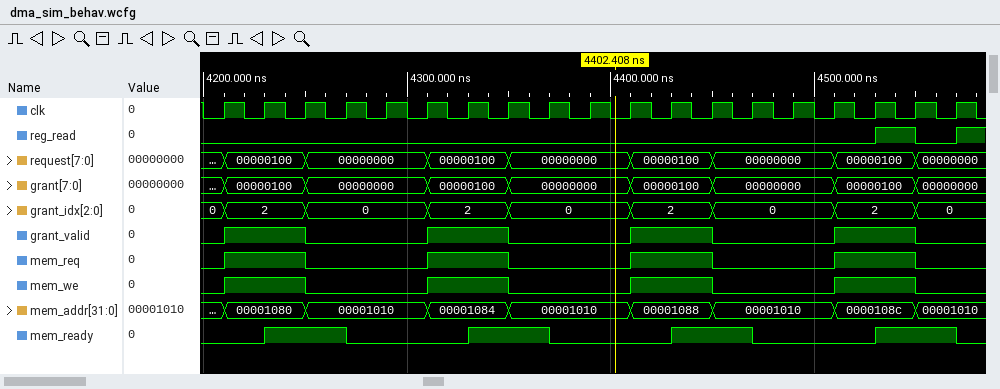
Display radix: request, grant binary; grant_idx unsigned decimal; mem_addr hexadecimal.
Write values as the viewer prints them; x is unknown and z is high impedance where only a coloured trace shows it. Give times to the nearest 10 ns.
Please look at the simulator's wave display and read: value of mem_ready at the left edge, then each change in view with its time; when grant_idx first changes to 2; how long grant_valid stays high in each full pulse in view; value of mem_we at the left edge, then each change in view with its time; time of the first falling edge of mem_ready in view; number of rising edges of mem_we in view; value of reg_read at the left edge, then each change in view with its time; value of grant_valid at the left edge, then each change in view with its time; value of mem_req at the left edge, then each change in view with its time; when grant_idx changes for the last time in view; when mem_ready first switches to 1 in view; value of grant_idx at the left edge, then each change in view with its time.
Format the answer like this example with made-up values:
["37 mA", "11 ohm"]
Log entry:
["0, 1 at 4230 ns, 0 at 4270 ns, 1 at 4330 ns, 0 at 4370 ns, 1 at 4430 ns, 0 at 4470 ns, 1 at 4530 ns, 0 at 4570 ns", "4210 ns", "40 ns, 40 ns, 40 ns, 40 ns", "0, 1 at 4210 ns, 0 at 4250 ns, 1 at 4310 ns, 0 at 4350 ns, 1 at 4410 ns, 0 at 4450 ns, 1 at 4510 ns, 0 at 4550 ns", "4270 ns", "4", "0, 1 at 4530 ns, 0 at 4550 ns, 1 at 4570 ns", "0, 1 at 4210 ns, 0 at 4250 ns, 1 at 4310 ns, 0 at 4350 ns, 1 at 4410 ns, 0 at 4450 ns, 1 at 4510 ns, 0 at 4550 ns", "0, 1 at 4210 ns, 0 at 4250 ns, 1 at 4310 ns, 0 at 4350 ns, 1 at 4410 ns, 0 at 4450 ns, 1 at 4510 ns, 0 at 4550 ns", "4550 ns", "4230 ns", "0, 2 at 4210 ns, 0 at 4250 ns, 2 at 4310 ns, 0 at 4350 ns, 2 at 4410 ns, 0 at 4450 ns, 2 at 4510 ns, 0 at 4550 ns"]
